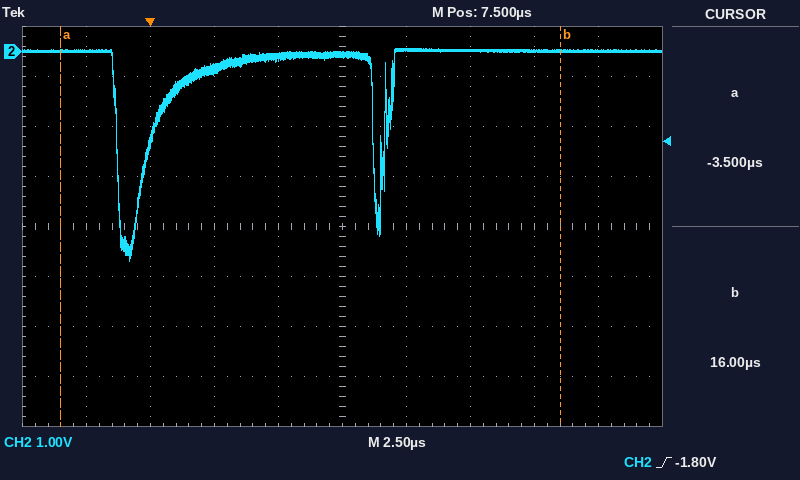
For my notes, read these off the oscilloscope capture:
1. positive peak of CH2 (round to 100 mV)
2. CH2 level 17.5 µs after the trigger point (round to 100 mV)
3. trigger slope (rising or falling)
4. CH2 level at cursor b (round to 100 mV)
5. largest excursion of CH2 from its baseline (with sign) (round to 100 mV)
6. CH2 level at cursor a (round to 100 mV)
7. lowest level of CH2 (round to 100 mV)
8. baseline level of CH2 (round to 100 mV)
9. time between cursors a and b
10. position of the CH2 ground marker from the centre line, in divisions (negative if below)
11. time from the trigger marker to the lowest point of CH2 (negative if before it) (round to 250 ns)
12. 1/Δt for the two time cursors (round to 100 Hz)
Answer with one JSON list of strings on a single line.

["100 mV", "0.0 V", "rising", "0.0 V", "-4.2 V", "0.0 V", "-4.2 V", "0.0 V", "19.50 µs", "+3.5 div", "-750 ns", "51.3 kHz"]
